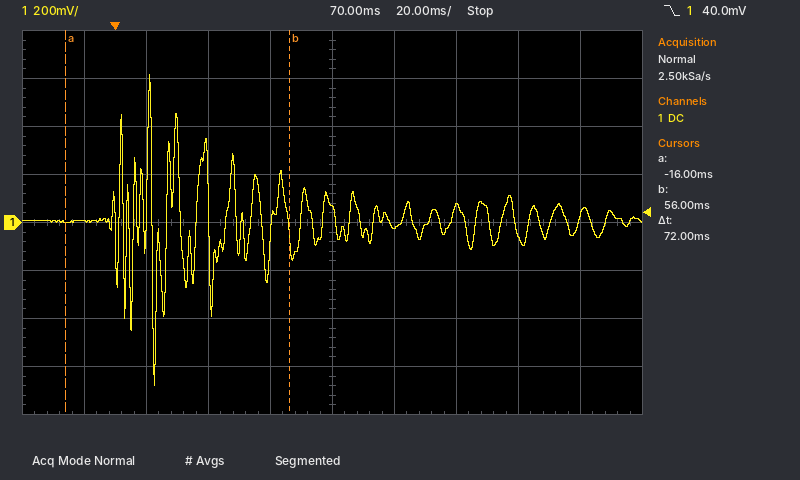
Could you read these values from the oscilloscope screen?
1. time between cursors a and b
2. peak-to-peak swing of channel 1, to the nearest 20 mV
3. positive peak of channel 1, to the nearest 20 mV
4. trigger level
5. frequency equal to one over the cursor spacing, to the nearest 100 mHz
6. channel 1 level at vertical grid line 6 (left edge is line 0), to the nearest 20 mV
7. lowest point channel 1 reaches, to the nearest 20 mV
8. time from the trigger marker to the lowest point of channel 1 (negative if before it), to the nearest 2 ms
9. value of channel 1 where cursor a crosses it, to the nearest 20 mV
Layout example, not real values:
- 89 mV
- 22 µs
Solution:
- 72 ms
- 1.30 V
- 620 mV
- 40.0 mV
- 13.9 Hz
- -20 mV
- -680 mV
- +12 ms
- 0 mV
